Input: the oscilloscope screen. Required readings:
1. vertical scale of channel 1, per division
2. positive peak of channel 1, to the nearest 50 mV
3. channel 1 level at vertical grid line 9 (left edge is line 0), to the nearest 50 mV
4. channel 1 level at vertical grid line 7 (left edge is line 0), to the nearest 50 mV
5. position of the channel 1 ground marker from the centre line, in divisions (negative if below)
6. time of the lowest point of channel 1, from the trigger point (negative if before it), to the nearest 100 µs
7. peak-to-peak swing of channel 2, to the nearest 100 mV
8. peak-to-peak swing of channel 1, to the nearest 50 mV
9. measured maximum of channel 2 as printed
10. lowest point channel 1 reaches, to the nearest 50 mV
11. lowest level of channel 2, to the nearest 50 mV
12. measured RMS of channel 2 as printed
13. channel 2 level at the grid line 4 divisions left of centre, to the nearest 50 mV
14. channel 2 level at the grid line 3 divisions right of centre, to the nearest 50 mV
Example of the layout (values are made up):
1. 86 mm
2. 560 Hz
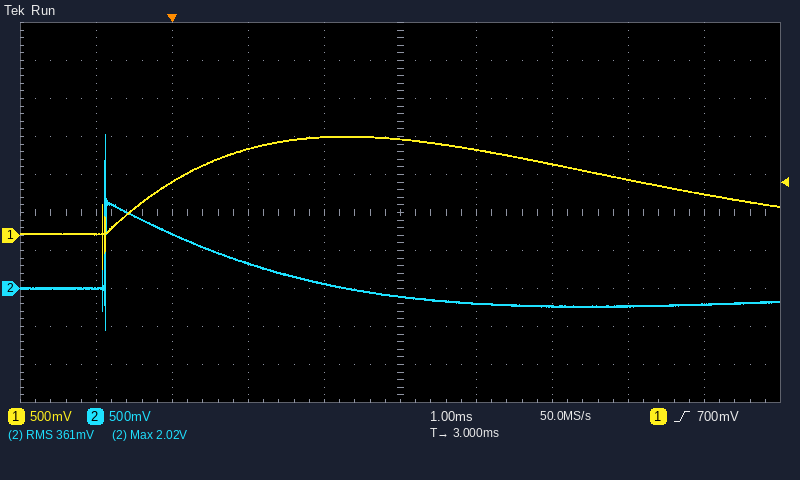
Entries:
1. 500 mV
2. 1.30 V
3. 550 mV
4. 950 mV
5. -0.6 div
6. -900 µs
7. 2.60 V
8. 1.75 V
9. 2.02 V
10. -450 mV
11. -550 mV
12. 361 mV
13. 0 mV
14. -250 mV
